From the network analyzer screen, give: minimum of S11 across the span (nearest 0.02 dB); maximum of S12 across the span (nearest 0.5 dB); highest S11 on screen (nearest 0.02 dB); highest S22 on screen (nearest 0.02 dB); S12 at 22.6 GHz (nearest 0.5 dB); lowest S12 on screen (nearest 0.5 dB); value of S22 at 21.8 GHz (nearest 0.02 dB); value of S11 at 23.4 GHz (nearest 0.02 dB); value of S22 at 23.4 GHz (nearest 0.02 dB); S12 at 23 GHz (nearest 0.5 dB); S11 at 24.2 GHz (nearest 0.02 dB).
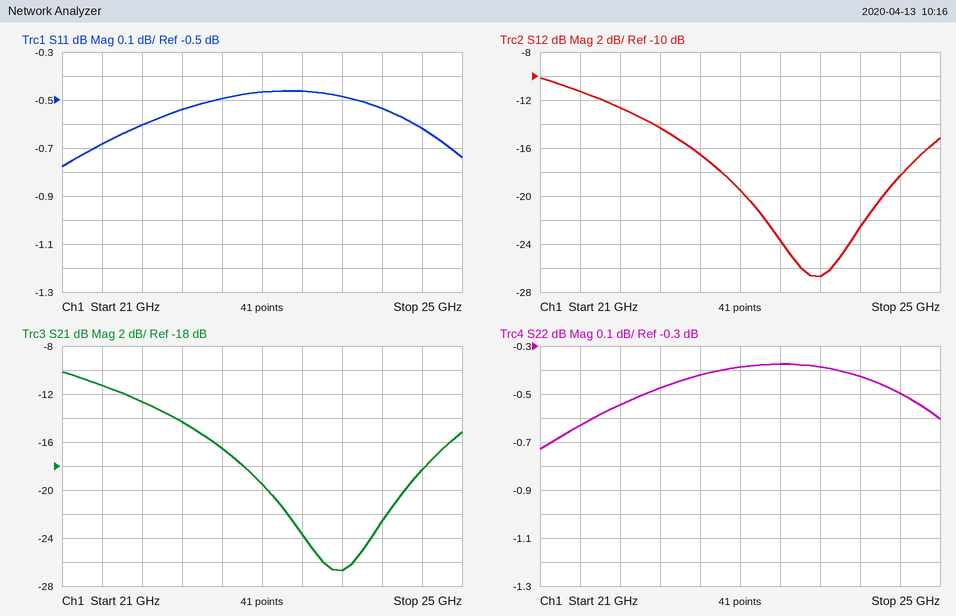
-0.78 dB
-10.0 dB
-0.46 dB
-0.38 dB
-16.5 dB
-26.5 dB
-0.54 dB
-0.46 dB
-0.38 dB
-19.5 dB
-0.54 dB
